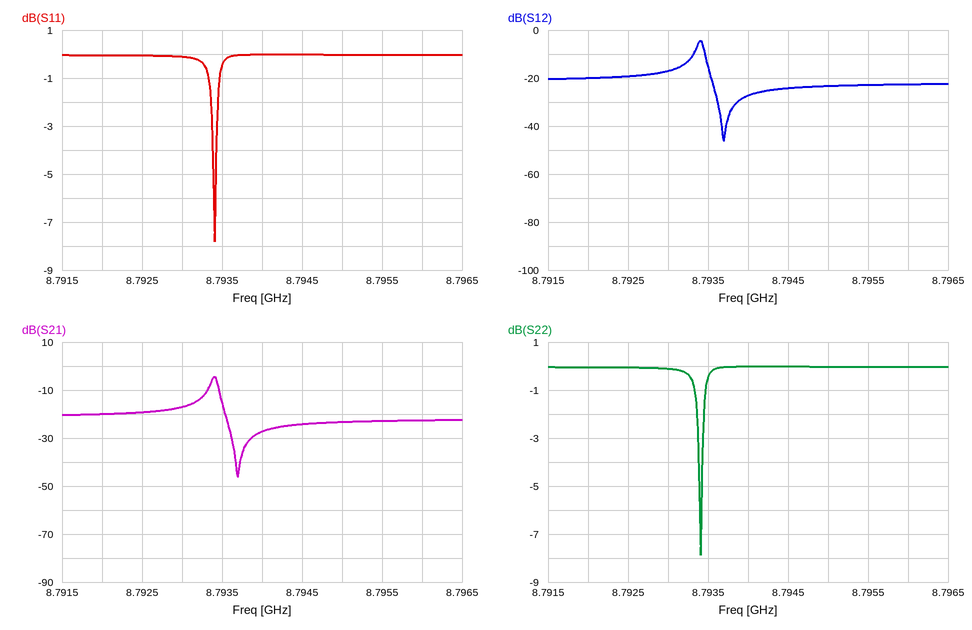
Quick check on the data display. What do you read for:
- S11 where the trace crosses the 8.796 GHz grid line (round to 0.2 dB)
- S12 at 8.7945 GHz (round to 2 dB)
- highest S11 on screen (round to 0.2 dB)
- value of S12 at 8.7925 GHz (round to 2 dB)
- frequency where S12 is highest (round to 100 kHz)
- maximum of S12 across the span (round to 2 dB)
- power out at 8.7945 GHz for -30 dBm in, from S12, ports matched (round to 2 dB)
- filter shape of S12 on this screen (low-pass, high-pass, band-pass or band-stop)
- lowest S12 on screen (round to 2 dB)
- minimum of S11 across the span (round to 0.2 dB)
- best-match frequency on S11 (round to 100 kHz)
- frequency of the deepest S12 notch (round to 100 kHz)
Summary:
0.0 dB
-24 dB
0.0 dB
-20 dB
8.7934 GHz
-4 dB
-54 dBm
band-pass
-46 dB
-7.8 dB
8.7934 GHz
8.7937 GHz
